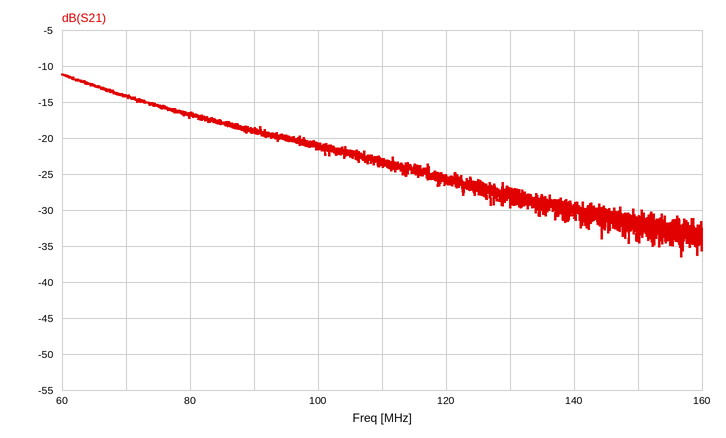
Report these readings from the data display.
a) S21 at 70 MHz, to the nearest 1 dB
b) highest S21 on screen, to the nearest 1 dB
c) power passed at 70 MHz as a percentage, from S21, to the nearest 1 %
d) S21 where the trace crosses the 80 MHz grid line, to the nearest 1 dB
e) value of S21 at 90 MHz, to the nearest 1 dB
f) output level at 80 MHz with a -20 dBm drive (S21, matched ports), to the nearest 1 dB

-14 dB
-11 dB
4 %
-17 dB
-19 dB
-37 dBm
